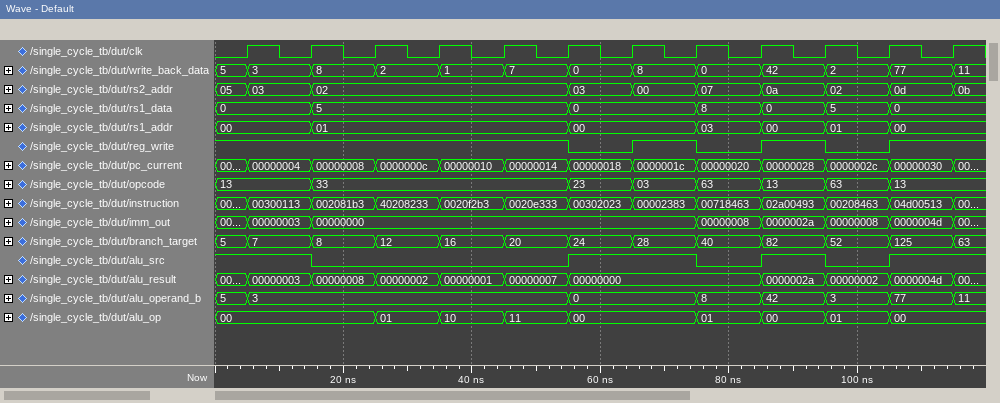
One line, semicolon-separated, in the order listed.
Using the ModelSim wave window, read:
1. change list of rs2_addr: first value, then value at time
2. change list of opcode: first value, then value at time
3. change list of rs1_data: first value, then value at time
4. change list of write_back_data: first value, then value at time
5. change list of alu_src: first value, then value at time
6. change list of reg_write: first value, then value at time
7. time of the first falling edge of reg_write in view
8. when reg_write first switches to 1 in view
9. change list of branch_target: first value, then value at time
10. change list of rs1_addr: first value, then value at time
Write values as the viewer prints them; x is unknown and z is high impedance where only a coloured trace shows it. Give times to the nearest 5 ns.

05, 03 at 5 ns, 02 at 15 ns, 03 at 55 ns, 00 at 65 ns, 07 at 75 ns, 0a at 85 ns, 02 at 95 ns, 0d at 105 ns, 0b at 115 ns; 13, 33 at 15 ns, 23 at 55 ns, 03 at 65 ns, 63 at 75 ns, 13 at 85 ns, 63 at 95 ns, 13 at 105 ns; 0, 5 at 15 ns, 0 at 55 ns, 8 at 75 ns, 0 at 85 ns, 5 at 95 ns, 0 at 105 ns; 5, 3 at 5 ns, 8 at 15 ns, 2 at 25 ns, 1 at 35 ns, 7 at 45 ns, 0 at 55 ns, 8 at 65 ns, 0 at 75 ns, 42 at 85 ns, 2 at 95 ns, 77 at 105 ns, 11 at 115 ns; 1, 0 at 15 ns, 1 at 55 ns, 0 at 75 ns, 1 at 85 ns, 0 at 95 ns, 1 at 105 ns; 1, 0 at 55 ns, 1 at 65 ns, 0 at 75 ns, 1 at 85 ns, 0 at 95 ns, 1 at 105 ns; 55 ns; 65 ns; 5, 7 at 5 ns, 8 at 15 ns, 12 at 25 ns, 16 at 35 ns, 20 at 45 ns, 24 at 55 ns, 28 at 65 ns, 40 at 75 ns, 82 at 85 ns, 52 at 95 ns, 125 at 105 ns, 63 at 115 ns; 00, 01 at 15 ns, 00 at 55 ns, 03 at 75 ns, 00 at 85 ns, 01 at 95 ns, 00 at 105 ns
